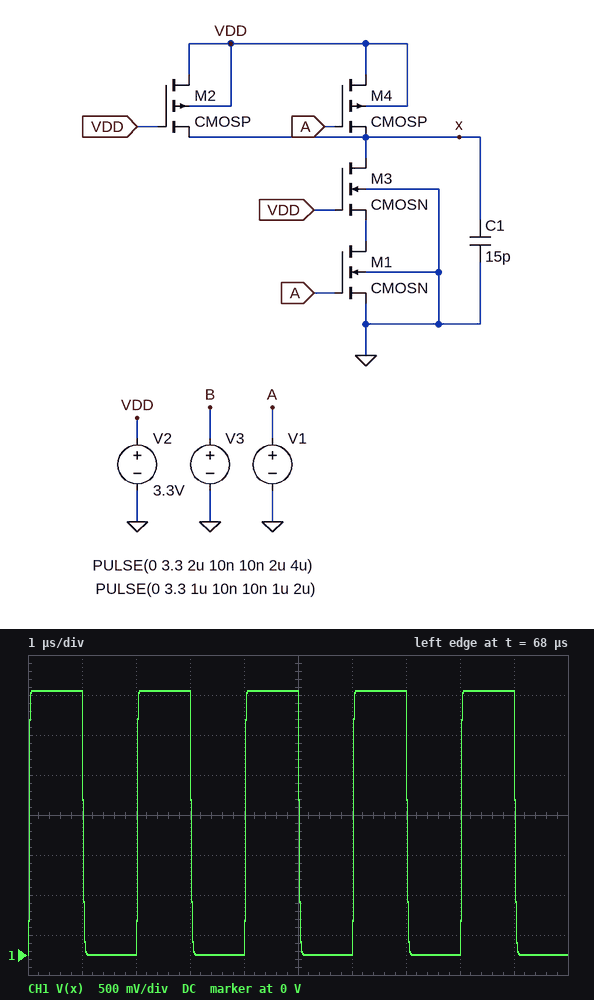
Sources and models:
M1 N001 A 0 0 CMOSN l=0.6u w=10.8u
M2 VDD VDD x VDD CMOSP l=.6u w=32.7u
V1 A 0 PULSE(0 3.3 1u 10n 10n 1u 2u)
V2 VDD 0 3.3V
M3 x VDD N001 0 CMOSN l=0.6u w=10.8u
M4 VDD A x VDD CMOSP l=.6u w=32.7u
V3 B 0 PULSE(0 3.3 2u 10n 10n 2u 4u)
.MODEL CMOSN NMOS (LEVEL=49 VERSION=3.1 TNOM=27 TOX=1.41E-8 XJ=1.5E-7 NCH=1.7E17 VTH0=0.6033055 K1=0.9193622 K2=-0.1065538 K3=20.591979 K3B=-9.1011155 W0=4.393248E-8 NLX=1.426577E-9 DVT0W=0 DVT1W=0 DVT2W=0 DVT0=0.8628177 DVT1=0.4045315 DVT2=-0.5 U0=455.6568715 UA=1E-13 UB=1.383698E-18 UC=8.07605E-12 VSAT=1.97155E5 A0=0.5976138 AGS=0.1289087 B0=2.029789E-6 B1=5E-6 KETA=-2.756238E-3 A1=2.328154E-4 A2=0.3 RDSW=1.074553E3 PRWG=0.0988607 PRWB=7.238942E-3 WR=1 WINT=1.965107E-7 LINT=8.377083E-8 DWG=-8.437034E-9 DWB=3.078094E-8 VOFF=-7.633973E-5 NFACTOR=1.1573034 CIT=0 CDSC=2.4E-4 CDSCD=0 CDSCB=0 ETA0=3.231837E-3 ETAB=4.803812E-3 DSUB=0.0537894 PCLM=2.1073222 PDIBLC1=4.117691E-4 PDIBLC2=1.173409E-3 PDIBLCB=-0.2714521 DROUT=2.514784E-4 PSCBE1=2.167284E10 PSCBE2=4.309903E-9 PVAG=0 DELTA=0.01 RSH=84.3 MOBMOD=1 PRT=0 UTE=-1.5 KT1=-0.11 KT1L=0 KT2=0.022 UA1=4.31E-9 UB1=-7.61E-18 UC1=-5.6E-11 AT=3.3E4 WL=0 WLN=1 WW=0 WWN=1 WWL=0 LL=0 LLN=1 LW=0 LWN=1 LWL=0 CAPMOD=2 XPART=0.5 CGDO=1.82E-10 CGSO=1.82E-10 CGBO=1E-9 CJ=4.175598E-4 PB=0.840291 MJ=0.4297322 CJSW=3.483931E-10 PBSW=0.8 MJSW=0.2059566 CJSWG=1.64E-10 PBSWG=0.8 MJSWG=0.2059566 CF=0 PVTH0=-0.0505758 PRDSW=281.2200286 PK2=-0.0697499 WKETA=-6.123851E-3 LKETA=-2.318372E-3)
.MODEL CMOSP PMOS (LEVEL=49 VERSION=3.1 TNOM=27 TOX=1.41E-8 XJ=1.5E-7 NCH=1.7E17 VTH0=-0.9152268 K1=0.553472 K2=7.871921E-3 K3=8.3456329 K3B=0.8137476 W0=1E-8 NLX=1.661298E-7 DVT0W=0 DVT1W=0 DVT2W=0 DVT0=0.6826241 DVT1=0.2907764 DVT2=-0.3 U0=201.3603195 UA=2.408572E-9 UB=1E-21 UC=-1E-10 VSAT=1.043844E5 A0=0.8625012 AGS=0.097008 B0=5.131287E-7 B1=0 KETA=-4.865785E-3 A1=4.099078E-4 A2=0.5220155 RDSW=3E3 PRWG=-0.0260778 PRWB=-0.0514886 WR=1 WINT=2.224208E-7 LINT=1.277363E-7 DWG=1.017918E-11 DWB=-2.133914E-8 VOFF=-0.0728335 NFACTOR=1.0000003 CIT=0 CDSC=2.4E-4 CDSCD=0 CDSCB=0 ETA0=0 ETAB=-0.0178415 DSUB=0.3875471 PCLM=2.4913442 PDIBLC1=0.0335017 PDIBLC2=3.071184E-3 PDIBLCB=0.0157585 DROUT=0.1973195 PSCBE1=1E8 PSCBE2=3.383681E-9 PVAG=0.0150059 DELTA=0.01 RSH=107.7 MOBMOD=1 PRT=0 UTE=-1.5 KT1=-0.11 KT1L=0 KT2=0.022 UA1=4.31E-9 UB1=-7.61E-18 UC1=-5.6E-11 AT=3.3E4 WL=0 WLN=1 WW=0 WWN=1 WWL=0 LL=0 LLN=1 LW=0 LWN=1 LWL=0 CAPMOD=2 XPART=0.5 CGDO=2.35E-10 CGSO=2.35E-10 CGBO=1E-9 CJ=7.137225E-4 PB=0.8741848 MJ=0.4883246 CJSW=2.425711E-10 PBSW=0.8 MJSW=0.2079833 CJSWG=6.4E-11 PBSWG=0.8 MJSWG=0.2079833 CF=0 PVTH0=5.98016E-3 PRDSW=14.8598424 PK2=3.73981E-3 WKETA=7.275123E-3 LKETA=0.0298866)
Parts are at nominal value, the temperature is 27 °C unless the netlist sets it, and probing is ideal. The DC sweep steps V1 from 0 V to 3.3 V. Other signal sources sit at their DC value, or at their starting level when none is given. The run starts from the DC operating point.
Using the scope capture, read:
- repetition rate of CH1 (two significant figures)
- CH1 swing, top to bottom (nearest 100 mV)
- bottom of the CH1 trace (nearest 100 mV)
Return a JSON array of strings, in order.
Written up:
["500 kHz", "3.3 V", "0 V"]
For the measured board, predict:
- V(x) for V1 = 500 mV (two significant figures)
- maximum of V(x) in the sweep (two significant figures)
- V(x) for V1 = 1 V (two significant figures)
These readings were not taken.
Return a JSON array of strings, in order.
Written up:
["3.3 V", "3.3 V", "3.2 V"]
